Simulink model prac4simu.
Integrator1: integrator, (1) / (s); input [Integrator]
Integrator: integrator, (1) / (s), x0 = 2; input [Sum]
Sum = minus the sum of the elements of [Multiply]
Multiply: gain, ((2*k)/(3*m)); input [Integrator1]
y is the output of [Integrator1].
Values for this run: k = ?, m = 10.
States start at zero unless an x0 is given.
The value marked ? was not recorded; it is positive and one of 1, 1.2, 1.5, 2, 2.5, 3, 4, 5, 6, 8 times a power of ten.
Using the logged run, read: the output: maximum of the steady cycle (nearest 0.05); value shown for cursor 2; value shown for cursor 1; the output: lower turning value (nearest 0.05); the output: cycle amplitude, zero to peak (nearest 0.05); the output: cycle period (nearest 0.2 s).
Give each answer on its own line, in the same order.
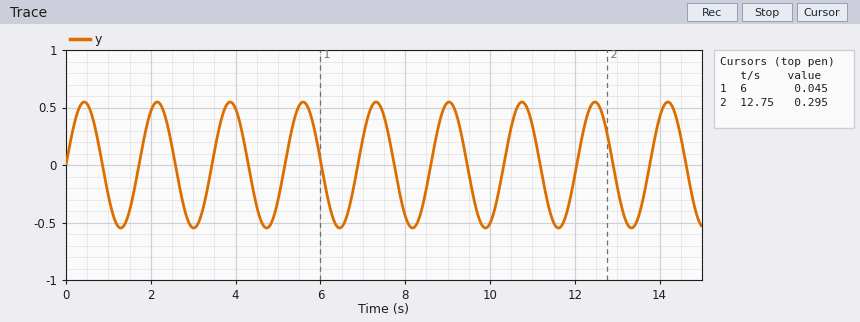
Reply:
0.55
0.295
0.045
-0.55
0.55
1.8 s
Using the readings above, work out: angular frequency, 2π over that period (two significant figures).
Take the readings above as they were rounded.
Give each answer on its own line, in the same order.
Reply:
3.5 rad/s
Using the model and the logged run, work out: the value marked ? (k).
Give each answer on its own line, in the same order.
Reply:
200
